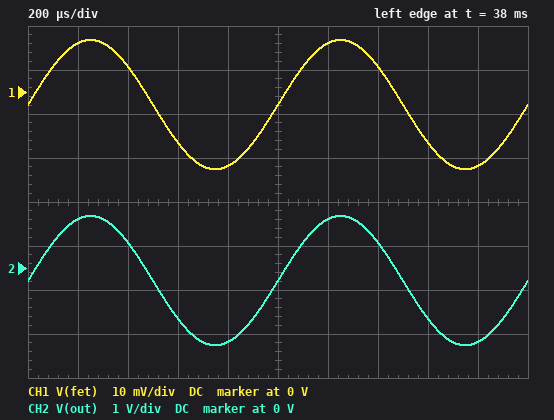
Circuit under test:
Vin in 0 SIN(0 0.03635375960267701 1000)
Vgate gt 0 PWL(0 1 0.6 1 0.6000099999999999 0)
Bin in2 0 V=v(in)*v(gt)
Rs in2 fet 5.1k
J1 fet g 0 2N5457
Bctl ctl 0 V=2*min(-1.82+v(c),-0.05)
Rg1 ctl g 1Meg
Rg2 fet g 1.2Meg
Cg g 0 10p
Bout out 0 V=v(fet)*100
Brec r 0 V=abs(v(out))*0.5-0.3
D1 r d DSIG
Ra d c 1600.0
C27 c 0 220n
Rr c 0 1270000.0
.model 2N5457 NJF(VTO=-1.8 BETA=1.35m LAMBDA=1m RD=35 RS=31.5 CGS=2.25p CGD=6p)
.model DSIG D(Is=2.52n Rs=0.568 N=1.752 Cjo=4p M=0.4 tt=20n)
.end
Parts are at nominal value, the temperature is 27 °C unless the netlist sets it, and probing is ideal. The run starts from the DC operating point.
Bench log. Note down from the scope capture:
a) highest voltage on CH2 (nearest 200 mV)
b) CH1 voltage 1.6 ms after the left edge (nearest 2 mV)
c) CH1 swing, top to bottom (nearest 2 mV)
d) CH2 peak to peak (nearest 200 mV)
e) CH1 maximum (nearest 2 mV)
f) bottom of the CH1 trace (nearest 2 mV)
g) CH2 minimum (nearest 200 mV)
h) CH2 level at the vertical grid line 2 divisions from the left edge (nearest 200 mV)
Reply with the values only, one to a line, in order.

1.2 V
-12 mV
30 mV
3.0 V
12 mV
-18 mV
-1.8 V
600 mV
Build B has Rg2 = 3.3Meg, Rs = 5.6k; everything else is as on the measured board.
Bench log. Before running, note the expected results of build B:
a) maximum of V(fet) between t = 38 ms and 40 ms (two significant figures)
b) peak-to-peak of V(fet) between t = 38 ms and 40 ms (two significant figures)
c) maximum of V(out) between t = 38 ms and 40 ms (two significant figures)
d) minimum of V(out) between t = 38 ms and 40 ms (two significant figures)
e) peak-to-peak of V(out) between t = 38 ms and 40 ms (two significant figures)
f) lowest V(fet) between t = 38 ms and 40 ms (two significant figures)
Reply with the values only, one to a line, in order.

26 mV
52 mV
2.6 V
-2.6 V
5.2 V
-26 mV
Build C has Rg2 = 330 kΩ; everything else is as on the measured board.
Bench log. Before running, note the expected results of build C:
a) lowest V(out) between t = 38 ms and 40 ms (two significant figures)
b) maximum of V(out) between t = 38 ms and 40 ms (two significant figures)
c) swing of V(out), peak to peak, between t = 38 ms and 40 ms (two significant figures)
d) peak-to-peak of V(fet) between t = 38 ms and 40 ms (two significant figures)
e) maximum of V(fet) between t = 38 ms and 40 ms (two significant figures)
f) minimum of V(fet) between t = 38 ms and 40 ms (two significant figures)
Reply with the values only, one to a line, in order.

-430 mV
190 mV
630 mV
6.3 mV
1.9 mV
-4.3 mV
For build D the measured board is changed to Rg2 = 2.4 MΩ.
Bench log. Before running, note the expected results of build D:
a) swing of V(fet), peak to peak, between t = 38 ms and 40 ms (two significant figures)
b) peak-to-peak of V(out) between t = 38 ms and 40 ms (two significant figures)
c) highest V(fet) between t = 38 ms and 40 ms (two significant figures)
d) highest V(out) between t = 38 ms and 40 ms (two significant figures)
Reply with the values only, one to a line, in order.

46 mV
4.6 V
22 mV
2.2 V
